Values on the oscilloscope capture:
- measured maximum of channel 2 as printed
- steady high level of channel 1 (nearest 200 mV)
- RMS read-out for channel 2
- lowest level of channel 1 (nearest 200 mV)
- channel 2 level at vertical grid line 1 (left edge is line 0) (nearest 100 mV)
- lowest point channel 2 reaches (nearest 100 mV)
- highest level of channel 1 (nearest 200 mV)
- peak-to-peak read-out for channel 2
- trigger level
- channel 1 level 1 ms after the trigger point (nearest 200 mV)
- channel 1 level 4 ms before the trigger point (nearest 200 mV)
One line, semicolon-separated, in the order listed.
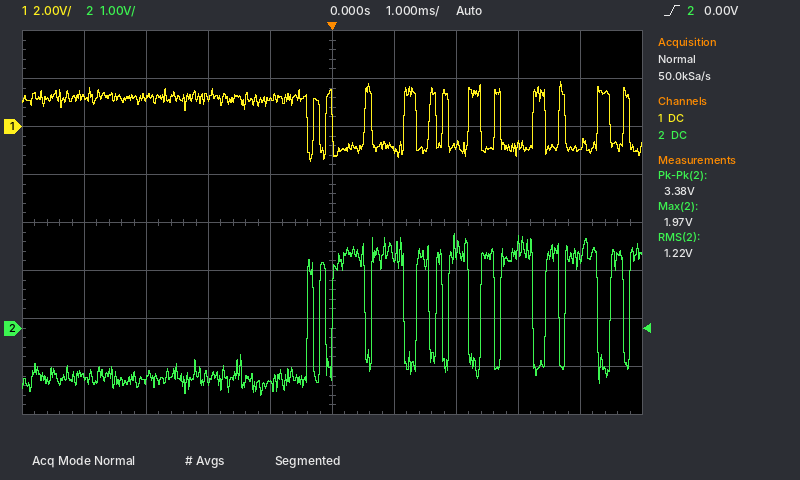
1.97 V; 1.2 V; 1.22 V; -1.4 V; -1.0 V; -1.4 V; 1.8 V; 3.38 V; 0.00 V; -1.0 V; 1.2 V
